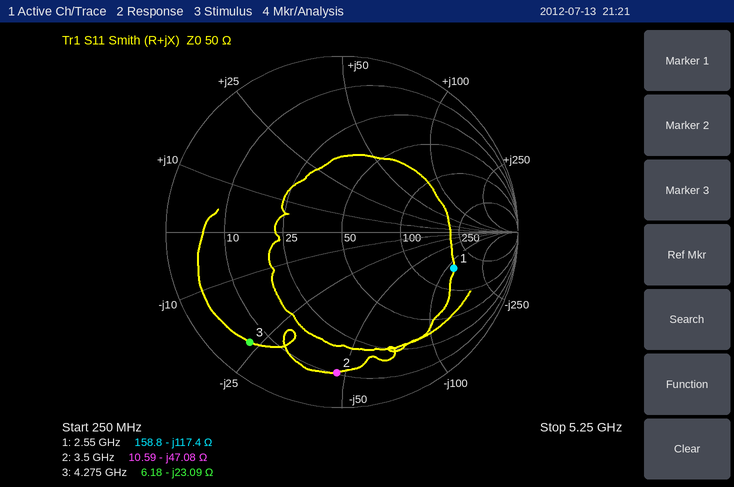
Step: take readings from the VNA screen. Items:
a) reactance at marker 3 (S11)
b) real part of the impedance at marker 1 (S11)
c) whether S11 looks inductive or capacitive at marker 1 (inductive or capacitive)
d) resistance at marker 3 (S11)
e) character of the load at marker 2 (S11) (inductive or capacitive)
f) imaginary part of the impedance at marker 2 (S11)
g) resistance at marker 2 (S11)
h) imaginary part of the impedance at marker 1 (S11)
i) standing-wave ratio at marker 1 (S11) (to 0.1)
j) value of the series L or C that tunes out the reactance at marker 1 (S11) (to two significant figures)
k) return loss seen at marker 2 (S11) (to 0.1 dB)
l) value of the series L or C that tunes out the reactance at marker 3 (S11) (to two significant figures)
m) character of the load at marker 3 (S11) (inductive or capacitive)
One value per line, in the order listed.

-23.09 Ω
158.8 Ω
capacitive
6.18 Ω
capacitive
-47.08 Ω
10.59 Ω
-117.4 Ω
5.0
7.3 nH
1.9 dB
860 pH
capacitive
